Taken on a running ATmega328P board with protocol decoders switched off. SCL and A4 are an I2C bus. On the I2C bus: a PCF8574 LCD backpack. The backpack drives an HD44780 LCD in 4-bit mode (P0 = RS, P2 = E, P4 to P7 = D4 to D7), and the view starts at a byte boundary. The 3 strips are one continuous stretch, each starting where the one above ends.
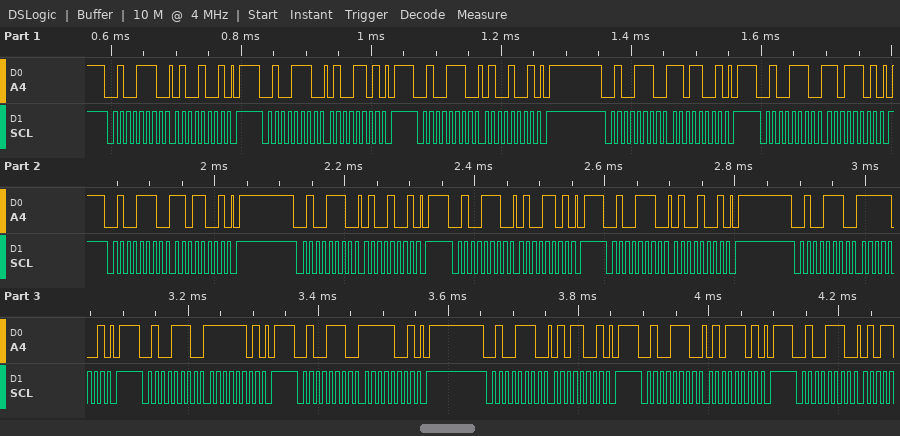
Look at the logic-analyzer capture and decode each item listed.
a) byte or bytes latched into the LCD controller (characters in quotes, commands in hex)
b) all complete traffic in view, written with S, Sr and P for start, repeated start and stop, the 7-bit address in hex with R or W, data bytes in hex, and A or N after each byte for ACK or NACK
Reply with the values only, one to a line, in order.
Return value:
'M' 'O'
S 27W A 49 A P S 27W A 4D A P S 27W A 49 A P S 27W A D9 A P S 27W A DD A P S 27W A D9 A P S 27W A 49 A P S 27W A 4D A P S 27W A 49 A P S 27W A F9 A P S 27W A FD A P S 27W A F9 A P S 27W A 59 A P S 27W A 5D A P S 27W A
